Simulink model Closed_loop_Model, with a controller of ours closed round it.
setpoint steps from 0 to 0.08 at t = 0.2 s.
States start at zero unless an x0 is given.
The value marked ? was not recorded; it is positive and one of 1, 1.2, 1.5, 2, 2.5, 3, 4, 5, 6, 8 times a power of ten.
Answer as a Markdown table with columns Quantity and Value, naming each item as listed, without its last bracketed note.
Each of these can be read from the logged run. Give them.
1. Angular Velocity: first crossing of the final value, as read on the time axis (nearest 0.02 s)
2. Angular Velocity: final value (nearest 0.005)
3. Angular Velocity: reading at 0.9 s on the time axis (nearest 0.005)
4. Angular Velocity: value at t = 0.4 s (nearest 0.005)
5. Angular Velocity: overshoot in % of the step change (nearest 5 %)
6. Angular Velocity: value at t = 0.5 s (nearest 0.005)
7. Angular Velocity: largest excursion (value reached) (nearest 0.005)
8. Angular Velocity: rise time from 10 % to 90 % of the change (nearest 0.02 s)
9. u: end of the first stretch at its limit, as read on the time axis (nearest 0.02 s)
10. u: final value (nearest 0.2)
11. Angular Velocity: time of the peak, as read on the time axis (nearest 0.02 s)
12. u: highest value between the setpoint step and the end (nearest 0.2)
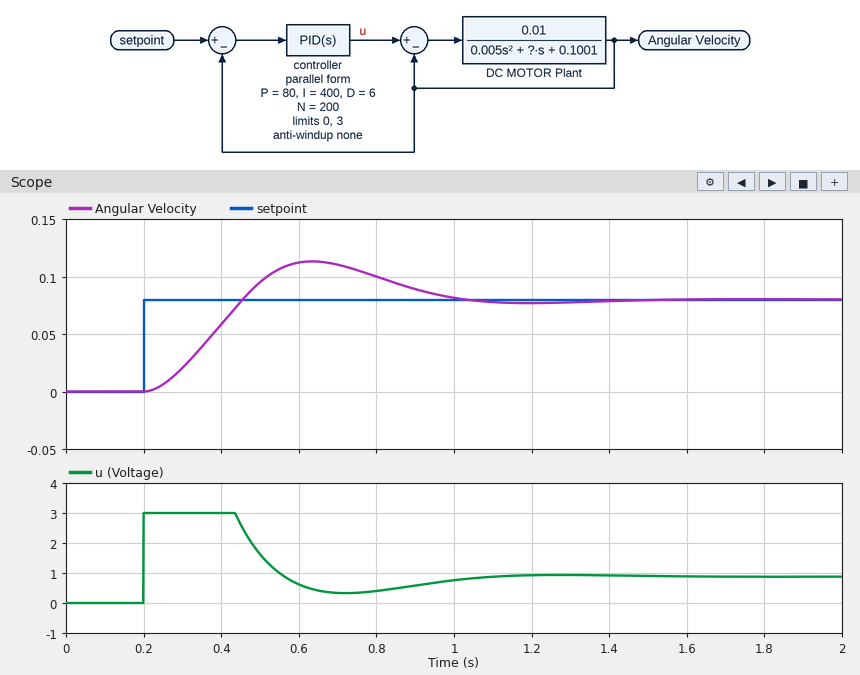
| Quantity | Value |
|---|---|
| Angular Velocity: first crossing of the final value, as read on the time axis | 0.46 s |
| Angular Velocity: final value | 0.080 |
| Angular Velocity: reading at 0.9 s on the time axis | 0.090 |
| Angular Velocity: value at t = 0.4 s | 0.060 |
| Angular Velocity: overshoot in % of the step change | 40 % |
| Angular Velocity: value at t = 0.5 s | 0.095 |
| Angular Velocity: largest excursion (value reached) | 0.115 |
| Angular Velocity: rise time from 10 % to 90 % of the change | 0.18 s |
| u: end of the first stretch at its limit, as read on the time axis | 0.44 s |
| u: final value | 0.8 |
| Angular Velocity: time of the peak, as read on the time axis | 0.64 s |
| u: highest value between the setpoint step and the end | 3.0 |
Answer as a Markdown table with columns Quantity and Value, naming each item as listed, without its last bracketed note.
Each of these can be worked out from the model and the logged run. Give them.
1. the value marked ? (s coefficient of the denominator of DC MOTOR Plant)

| Quantity | Value |
|---|---|
| the value marked ? | 0.06 |
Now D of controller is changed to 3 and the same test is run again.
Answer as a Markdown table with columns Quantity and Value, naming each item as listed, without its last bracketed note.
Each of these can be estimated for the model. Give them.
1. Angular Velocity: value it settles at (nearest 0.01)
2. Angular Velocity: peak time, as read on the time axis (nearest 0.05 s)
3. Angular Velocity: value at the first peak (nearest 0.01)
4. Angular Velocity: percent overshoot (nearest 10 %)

| Quantity | Value |
|---|---|
| Angular Velocity: value it settles at | 0.08 |
| Angular Velocity: peak time, as read on the time axis | 0.60 s |
| Angular Velocity: value at the first peak | 0.12 |
| Angular Velocity: percent overshoot | 50 % |
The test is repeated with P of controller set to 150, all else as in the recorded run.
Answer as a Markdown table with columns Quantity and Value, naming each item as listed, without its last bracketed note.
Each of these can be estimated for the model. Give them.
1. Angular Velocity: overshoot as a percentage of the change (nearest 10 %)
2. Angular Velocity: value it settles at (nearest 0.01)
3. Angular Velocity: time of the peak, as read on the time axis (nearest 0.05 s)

| Quantity | Value |
|---|---|
| Angular Velocity: overshoot as a percentage of the change | 30 % |
| Angular Velocity: value it settles at | 0.08 |
| Angular Velocity: time of the peak, as read on the time axis | 0.60 s |
